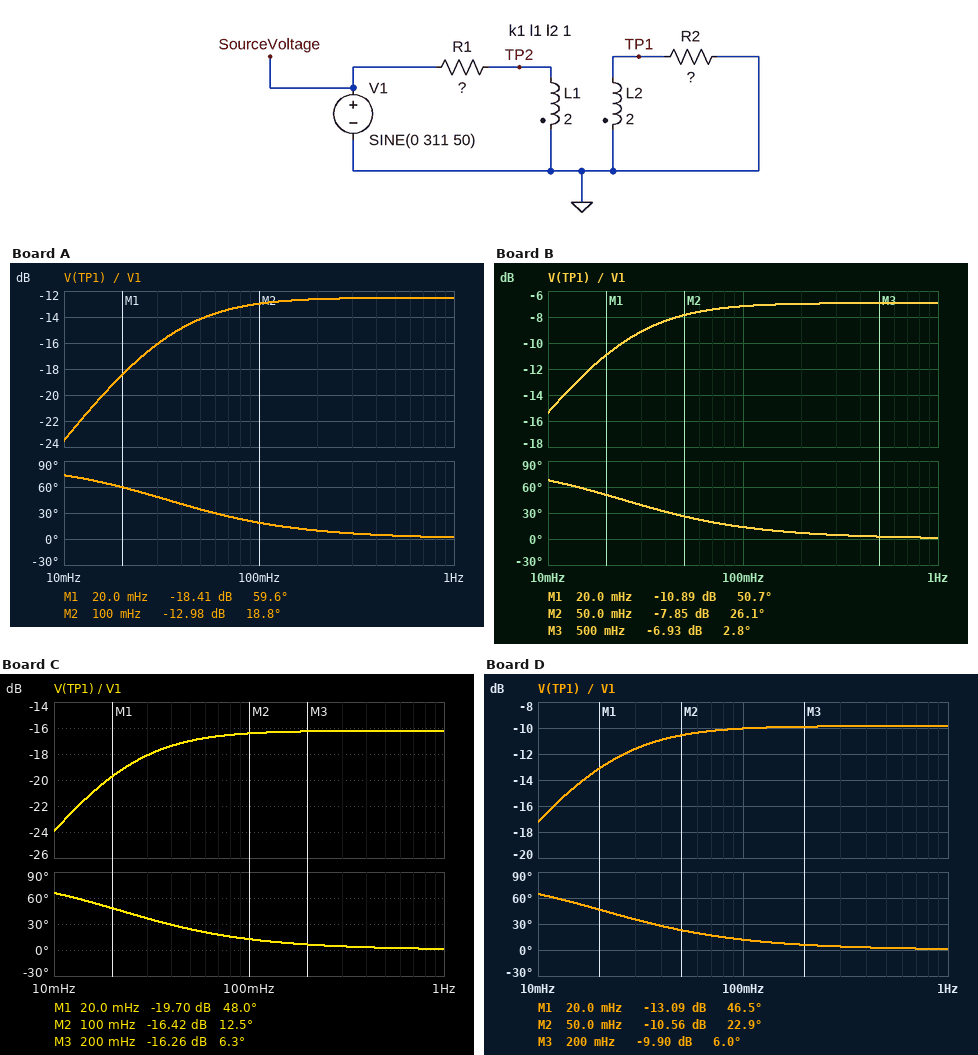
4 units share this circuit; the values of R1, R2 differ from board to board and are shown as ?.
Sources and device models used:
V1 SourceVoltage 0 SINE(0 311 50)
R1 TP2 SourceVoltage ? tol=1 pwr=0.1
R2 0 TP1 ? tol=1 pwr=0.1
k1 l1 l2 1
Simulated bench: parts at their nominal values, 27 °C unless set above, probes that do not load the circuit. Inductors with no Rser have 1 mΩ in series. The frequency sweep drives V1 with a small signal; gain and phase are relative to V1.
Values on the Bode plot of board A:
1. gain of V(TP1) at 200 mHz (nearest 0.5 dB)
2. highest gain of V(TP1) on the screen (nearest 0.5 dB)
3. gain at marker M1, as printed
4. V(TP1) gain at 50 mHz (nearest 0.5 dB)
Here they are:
-12.5 dB
-12.5 dB
-18.41 dB
-14.0 dB
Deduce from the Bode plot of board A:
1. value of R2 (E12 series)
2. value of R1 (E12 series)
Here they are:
0.56 Ω
1.8 Ω
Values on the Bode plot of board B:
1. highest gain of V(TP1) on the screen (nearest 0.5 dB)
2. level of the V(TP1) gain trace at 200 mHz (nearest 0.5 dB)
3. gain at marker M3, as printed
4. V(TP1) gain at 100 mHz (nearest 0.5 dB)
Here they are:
-7.0 dB
-7.0 dB
-6.93 dB
-7.0 dB
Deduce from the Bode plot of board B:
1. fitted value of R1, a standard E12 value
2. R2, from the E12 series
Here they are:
0.68 Ω
0.56 Ω
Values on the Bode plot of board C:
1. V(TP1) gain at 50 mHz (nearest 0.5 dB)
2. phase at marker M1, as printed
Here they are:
-17.0 dB
48.0 deg
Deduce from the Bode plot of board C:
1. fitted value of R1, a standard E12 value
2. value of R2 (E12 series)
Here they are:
1.8 Ω
0.33 Ω
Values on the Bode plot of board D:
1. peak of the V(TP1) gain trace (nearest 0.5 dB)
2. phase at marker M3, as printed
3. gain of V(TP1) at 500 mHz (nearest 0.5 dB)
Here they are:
-10.0 dB
6.0 deg
-10.0 dB
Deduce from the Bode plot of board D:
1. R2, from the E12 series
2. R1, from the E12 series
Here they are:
0.39 Ω
0.82 Ω
